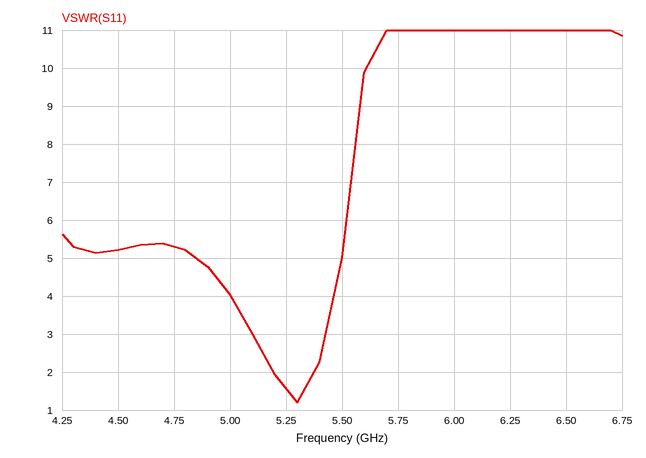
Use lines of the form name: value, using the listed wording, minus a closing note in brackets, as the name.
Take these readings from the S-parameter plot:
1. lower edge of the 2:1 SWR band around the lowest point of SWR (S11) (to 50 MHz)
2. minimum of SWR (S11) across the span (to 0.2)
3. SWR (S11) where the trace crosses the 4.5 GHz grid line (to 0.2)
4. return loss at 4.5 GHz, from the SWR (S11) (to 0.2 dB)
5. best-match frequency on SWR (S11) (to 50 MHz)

lower edge of the 2:1 SWR band around the lowest point of SWR (S11): 5.20 GHz
minimum of SWR (S11) across the span: 1.2
SWR (S11) where the trace crosses the 4.5 GHz grid line: 5.2
return loss at 4.5 GHz, from the SWR (S11): 3.4 dB
best-match frequency on SWR (S11): 5.30 GHz
